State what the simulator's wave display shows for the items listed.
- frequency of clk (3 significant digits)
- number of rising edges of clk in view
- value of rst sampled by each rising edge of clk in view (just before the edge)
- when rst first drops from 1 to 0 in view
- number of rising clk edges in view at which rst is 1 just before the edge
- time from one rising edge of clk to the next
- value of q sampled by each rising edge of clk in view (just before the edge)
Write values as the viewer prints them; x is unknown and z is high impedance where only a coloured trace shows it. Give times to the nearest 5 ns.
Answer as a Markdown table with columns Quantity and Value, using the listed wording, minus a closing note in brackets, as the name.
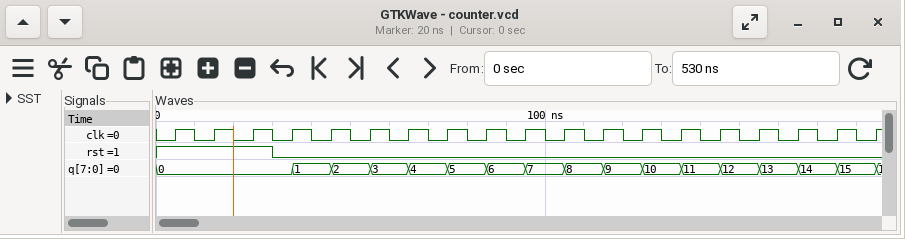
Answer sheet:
| Quantity | Value |
|---|---|
| frequency of clk | 100 MHz |
| number of rising edges of clk in view | 19 |
| value of rst sampled by each rising edge of clk in view | 1 1 1 0 0 0 0 0 0 0 0 0 0 0 0 0 0 0 0 |
| when rst first drops from 1 to 0 in view | 30 ns |
| number of rising clk edges in view at which rst is 1 just before the edge | 3 |
| time from one rising edge of clk to the next | 10 ns |
| value of q sampled by each rising edge of clk in view | 0, 0, 0, 0, 1, 2, 3, 4, 5, 6, 7, 8, 9, 10, 11, 12, 13, 14, 15 |
